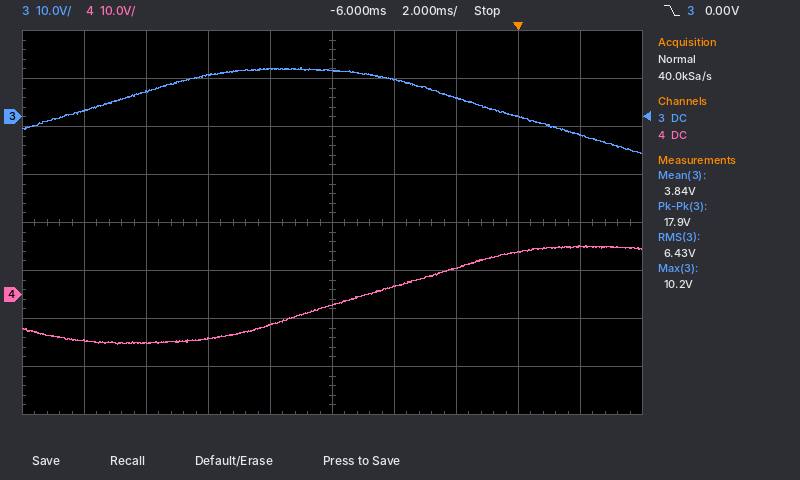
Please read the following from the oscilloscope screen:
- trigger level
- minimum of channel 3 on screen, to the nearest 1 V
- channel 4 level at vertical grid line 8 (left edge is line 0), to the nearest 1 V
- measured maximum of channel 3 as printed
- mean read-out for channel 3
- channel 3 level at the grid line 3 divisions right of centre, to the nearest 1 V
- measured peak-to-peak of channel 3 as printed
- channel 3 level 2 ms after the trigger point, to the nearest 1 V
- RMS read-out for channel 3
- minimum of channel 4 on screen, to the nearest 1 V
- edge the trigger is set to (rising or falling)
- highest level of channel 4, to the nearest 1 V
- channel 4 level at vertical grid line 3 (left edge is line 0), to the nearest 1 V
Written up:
0.00 V
-8 V
9 V
10.2 V
3.84 V
0 V
17.9 V
-4 V
6.43 V
-10 V
falling
10 V
-9 V
